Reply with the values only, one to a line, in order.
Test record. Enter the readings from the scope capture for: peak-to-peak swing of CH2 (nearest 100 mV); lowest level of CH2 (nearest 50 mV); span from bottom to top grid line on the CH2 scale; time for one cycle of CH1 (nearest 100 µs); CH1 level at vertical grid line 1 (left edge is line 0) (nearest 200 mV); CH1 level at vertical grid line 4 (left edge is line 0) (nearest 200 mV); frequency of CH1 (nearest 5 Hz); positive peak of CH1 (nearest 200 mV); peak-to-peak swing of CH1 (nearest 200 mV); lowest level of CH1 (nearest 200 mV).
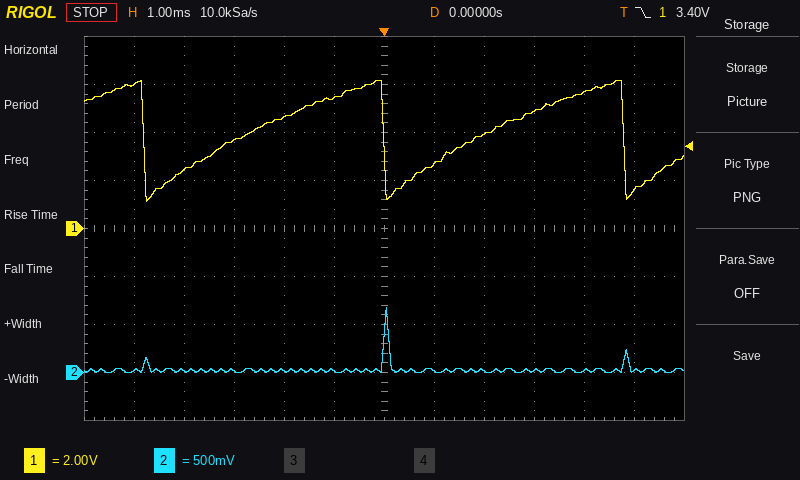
700 mV
0 mV
4 V
4.8 ms
6.0 V
4.6 V
210 Hz
6.2 V
5.0 V
1.2 V
